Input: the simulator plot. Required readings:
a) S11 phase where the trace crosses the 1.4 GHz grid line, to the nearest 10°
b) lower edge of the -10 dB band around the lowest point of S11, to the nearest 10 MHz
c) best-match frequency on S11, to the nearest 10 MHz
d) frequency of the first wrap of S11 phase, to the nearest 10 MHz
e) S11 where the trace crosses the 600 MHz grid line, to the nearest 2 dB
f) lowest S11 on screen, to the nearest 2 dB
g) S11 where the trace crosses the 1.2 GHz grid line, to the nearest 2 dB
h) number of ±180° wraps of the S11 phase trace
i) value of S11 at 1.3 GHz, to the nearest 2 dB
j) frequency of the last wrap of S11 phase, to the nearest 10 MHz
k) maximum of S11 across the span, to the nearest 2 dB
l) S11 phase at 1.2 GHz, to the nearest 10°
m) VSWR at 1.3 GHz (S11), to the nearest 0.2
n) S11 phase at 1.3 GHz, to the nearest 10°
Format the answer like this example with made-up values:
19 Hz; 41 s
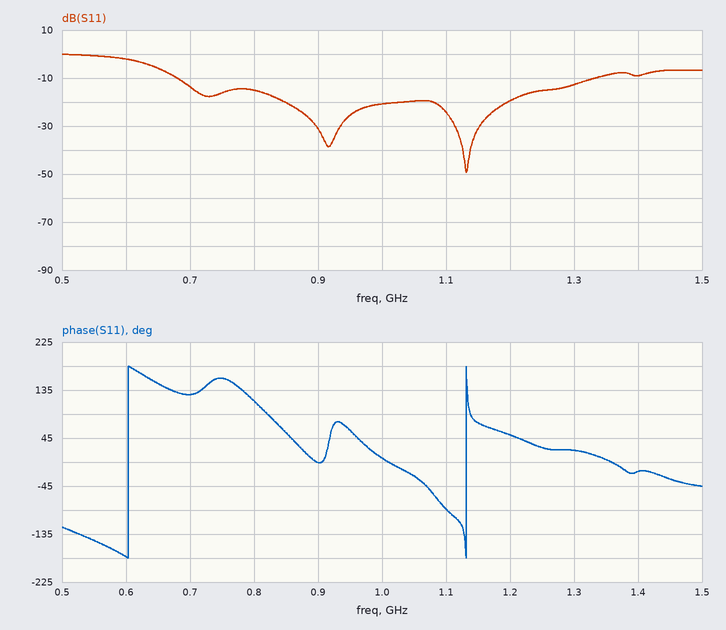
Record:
-20°; 680 MHz; 1.13 GHz; 600 MHz; -2 dB; -50 dB; -20 dB; 2; -12 dB; 1.13 GHz; 0 dB; 50°; 1.6; 20°
